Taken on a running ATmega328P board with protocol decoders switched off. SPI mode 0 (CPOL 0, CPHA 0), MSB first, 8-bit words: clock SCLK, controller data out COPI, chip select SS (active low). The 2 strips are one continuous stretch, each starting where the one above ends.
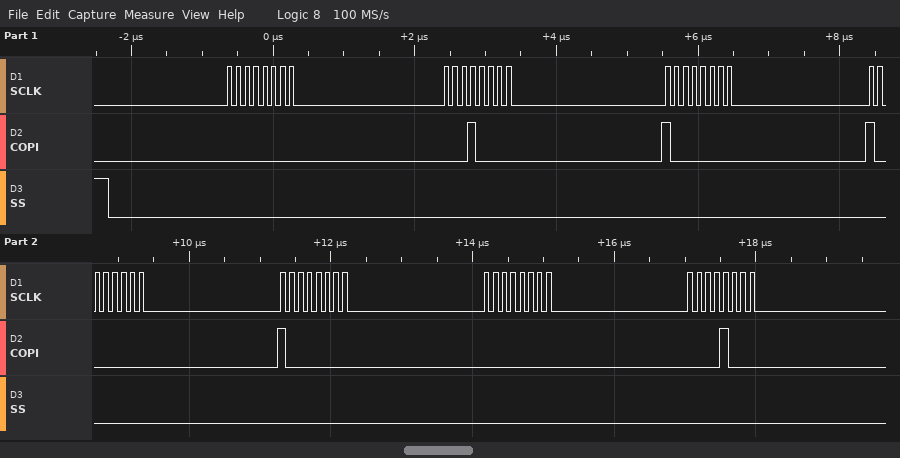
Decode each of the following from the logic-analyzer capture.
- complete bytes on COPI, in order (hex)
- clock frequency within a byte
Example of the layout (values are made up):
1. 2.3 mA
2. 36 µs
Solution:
1. 0x00 0x10 0x80 0x80 0x80 0x00 0x08
2. 8 MHz
